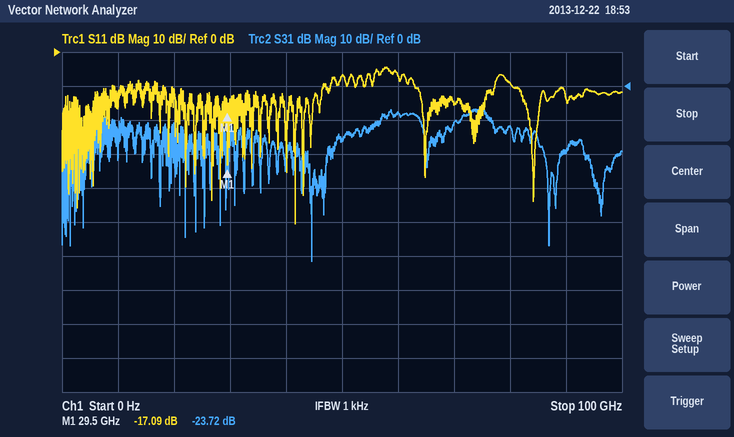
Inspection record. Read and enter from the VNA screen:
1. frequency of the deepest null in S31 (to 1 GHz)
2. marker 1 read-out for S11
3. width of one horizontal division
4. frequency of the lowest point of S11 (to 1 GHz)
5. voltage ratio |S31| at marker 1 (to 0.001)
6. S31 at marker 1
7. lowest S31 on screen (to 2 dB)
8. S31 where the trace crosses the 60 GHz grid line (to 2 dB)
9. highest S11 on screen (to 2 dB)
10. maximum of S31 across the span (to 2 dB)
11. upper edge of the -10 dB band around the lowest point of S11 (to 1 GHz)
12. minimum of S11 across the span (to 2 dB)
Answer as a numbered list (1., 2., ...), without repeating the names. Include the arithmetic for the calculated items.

1. 45 GHz
2. -17.09 dB
3. 10 GHz
4. 42 GHz
5. 10^(-23.72/20) ≈ 0.065
6. -23.72 dB
7. -52 dB
8. -8 dB
9. -4 dB
10. -6 dB
11. 47 GHz
12. -50 dB
